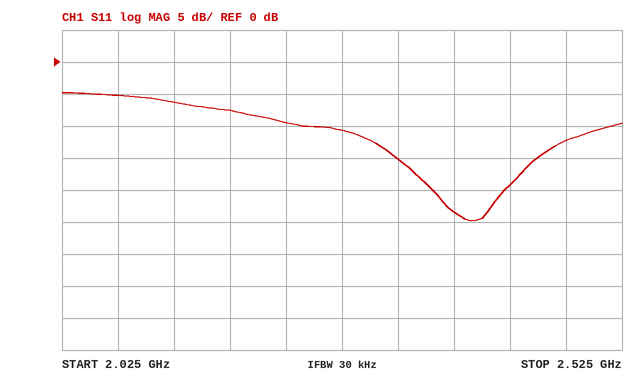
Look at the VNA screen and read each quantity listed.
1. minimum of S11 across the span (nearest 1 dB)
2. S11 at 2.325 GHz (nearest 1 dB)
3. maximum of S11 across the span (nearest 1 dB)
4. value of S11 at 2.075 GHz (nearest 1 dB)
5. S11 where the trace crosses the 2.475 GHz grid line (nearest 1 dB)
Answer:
-25 dB
-15 dB
-5 dB
-5 dB
-12 dB
